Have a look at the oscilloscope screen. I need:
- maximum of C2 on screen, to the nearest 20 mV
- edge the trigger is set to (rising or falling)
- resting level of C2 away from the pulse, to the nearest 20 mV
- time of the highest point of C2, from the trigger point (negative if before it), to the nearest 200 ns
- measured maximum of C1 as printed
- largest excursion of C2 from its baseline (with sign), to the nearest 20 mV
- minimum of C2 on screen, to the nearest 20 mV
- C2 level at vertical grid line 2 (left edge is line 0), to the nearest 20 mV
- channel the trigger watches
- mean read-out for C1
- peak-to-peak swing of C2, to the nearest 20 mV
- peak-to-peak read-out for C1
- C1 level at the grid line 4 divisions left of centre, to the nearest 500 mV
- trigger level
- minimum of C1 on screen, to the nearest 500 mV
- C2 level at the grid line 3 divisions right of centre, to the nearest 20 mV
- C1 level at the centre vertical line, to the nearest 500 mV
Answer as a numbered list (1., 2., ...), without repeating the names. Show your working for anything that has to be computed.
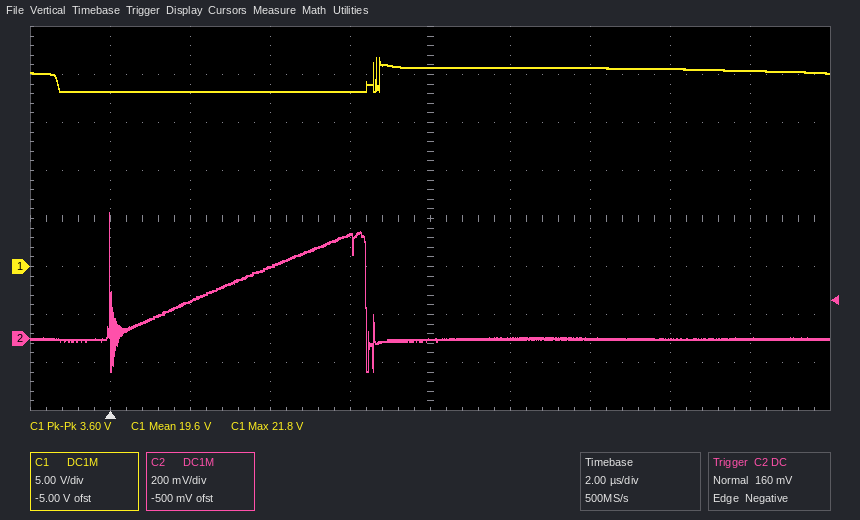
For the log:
1. 520 mV
2. falling
3. 0 mV
4. 0.0 µs
5. 21.8 V
6. 520 mV − (0 mV) = +520 mV
7. -140 mV
8. 160 mV
9. C2
10. 19.6 V
11. 520 mV − (-140 mV) = 660 mV
12. 3.60 V
13. 18.0 V
14. 160 mV
15. 18.0 V
16. 0 mV
17. 20.5 V
